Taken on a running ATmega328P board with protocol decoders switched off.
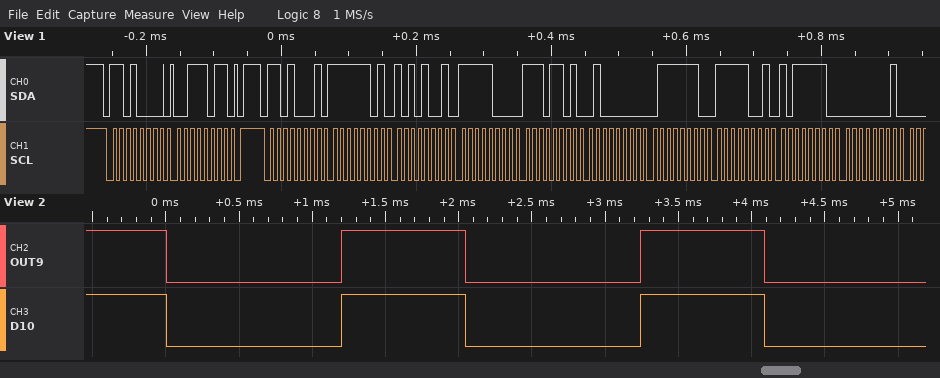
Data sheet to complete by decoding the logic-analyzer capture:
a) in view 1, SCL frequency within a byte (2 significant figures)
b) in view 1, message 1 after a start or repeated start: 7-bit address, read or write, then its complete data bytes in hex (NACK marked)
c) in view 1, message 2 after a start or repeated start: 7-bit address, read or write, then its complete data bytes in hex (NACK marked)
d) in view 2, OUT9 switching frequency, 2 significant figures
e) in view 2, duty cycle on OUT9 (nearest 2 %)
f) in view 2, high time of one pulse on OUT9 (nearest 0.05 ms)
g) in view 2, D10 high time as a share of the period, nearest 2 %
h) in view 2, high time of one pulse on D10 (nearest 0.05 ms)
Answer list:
100 kHz
0x68 write: 3B
0x68 read: FD A9 F8 ED 40 7E F9 BE 01
490 Hz
42 %
0.85 ms
42 %
0.85 ms
